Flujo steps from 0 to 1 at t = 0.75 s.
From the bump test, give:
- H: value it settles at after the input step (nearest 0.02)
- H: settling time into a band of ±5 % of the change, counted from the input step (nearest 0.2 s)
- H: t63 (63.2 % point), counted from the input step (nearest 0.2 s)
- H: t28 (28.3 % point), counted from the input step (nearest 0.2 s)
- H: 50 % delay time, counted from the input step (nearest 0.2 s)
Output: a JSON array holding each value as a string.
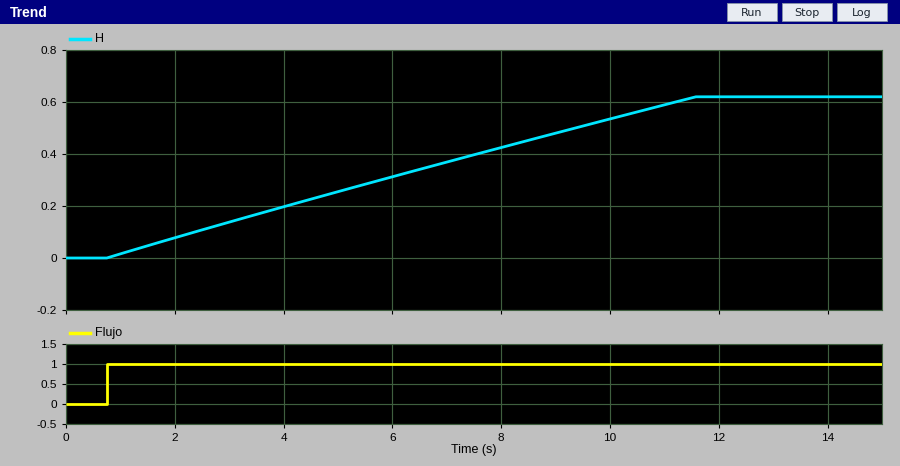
["0.62", "10.2 s", "6.6 s", "2.8 s", "5.2 s"]
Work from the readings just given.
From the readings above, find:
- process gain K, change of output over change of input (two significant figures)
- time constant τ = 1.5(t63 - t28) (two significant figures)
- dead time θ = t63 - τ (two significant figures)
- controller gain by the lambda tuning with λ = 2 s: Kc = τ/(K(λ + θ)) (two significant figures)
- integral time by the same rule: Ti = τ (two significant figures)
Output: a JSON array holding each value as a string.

["0.62", "5.7 s", "0.90 s", "3.2", "5.7 s"]
